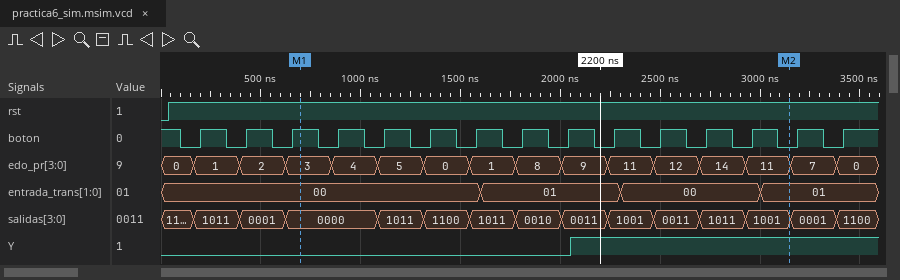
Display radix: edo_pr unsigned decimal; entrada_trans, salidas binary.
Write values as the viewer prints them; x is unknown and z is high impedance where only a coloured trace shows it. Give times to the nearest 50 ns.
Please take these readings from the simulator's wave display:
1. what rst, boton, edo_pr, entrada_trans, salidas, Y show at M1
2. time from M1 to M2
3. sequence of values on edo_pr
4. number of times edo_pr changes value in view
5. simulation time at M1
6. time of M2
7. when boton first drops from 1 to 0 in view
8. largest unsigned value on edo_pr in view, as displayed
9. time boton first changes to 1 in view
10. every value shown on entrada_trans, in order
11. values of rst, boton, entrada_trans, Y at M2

rst=1, boton=1, edo_pr=3, entrada_trans=00, salidas=0000, Y=0
2450 ns
0, 1, 2, 3, 4, 5, 0, 1, 8, 9, 11, 12, 14, 11, 7, 0
15
700 ns
3150 ns
100 ns
14
200 ns
00, 01, 00, 01
rst=1, boton=0, entrada_trans=01, Y=1
